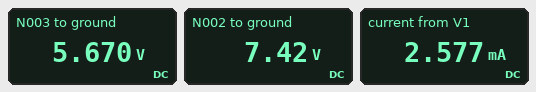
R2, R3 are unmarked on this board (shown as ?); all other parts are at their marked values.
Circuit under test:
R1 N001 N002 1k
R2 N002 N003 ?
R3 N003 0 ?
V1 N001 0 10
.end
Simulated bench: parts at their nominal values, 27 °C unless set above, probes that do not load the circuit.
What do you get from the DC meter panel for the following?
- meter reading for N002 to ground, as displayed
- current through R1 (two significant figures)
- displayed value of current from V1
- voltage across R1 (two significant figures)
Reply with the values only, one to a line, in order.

7.42 V
2.6 mA
2.577 mA
2.6 V
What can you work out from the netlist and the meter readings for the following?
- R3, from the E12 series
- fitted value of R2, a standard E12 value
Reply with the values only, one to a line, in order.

2.2 kΩ
680 Ω
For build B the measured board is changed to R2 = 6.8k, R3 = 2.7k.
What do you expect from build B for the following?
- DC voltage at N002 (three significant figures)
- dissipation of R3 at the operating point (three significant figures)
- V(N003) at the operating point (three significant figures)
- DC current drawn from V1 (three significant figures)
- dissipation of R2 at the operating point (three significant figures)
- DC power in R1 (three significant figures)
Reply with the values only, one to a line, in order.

9.05 V
2.45 mW
2.57 V
952 µA
6.17 mW
907 µW
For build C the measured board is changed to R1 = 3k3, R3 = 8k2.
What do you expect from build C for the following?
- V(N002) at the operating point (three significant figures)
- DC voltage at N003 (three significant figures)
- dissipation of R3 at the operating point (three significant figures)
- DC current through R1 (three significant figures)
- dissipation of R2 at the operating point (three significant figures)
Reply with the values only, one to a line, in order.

7.29 V
6.73 V
5.53 mW
821 µA
458 µW
